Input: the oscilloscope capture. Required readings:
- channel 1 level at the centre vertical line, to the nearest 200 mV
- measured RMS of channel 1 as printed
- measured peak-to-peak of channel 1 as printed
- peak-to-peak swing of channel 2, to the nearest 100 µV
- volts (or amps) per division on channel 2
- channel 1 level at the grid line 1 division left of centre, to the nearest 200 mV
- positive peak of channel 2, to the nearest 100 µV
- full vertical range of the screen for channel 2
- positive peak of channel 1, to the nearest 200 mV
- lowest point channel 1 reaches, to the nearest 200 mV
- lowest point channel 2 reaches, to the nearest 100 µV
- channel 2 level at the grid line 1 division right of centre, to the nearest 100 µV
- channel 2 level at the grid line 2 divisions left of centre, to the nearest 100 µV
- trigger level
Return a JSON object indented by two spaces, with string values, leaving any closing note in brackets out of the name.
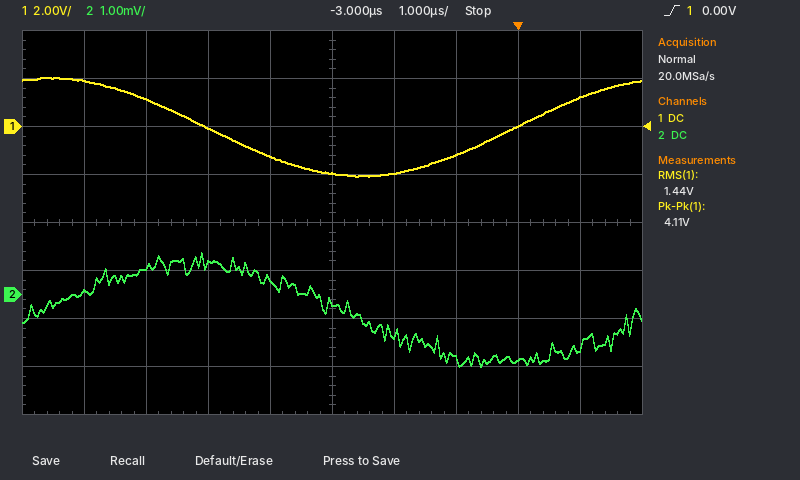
{
  "channel 1 level at the centre vertical line, to the nearest 200 mV": "-2.0 V",
  "measured RMS of channel 1 as printed": "1.44 V",
  "measured peak-to-peak of channel 1 as printed": "4.11 V",
  "peak-to-peak swing of channel 2, to the nearest 100 µV": "2.4 mV",
  "volts (or amps) per division on channel 2": "1 mV",
  "channel 1 level at the grid line 1 division left of centre, to the nearest 200 mV": "-1.2 V",
  "positive peak of channel 2, to the nearest 100 µV": "900 µV",
  "full vertical range of the screen for channel 2": "8 mV",
  "positive peak of channel 1, to the nearest 200 mV": "2.0 V",
  "lowest point channel 1 reaches, to the nearest 200 mV": "-2.0 V",
  "lowest point channel 2 reaches, to the nearest 100 µV": "-1.5 mV",
  "channel 2 level at the grid line 1 division right of centre, to the nearest 100 µV": "-800 µV",
  "channel 2 level at the grid line 2 divisions left of centre, to the nearest 100 µV": "600 µV",
  "trigger level": "0.00 V"
}
